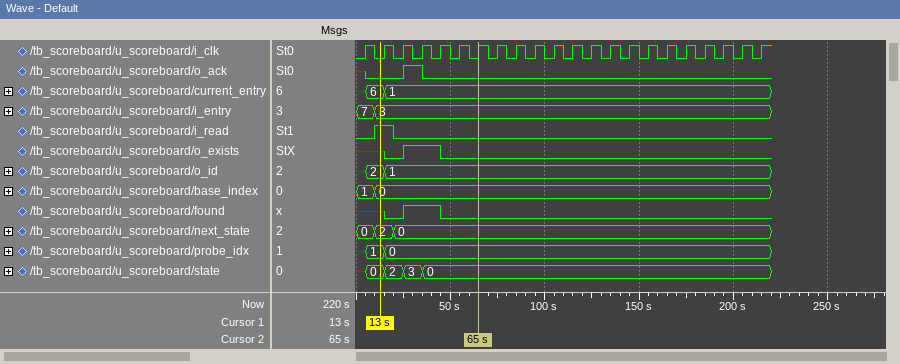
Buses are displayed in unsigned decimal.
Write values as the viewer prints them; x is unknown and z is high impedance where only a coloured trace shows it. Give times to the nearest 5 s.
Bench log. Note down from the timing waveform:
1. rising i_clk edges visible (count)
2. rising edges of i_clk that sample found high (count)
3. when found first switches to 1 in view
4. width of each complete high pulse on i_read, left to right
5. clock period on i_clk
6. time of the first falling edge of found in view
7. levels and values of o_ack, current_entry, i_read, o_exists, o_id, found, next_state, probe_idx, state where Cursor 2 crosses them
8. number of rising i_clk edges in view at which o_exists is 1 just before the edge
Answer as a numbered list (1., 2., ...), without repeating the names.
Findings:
1. 22
2. 2
3. 25 s
4. 10 s
5. 10 s
6. 45 s
7. o_ack=0, current_entry=1, i_read=0, o_exists=0, o_id=1, found=0, next_state=0, probe_idx=0, state=0
8. 2
